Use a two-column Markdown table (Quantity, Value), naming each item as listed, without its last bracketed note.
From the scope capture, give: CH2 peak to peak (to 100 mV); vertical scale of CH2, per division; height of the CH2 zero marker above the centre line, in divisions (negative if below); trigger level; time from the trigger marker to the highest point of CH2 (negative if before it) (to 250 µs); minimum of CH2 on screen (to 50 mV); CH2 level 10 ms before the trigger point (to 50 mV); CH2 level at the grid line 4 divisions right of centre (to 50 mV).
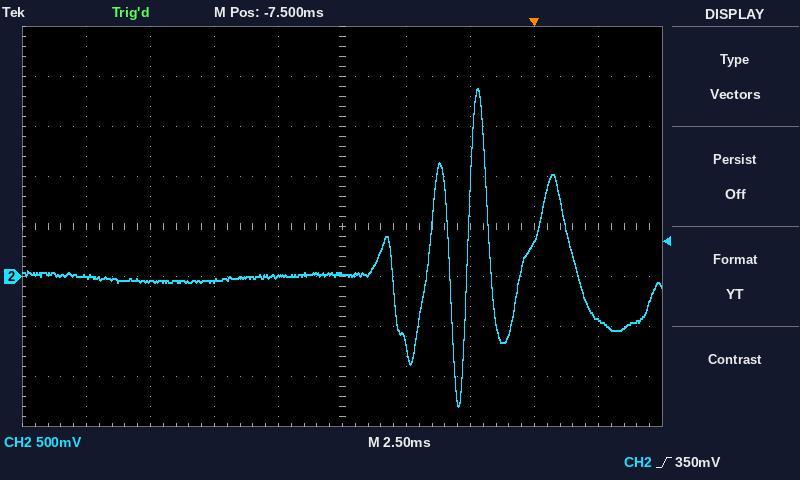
| Quantity | Value |
|---|---|
| CH2 peak to peak | 3.20 V |
| vertical scale of CH2, per division | 500 mV |
| height of the CH2 zero marker above the centre line, in divisions | -1.0 div |
| trigger level | 350 mV |
| time from the trigger marker to the highest point of CH2 (negative if before it) | -2.25 ms |
| minimum of CH2 on screen | -1.30 V |
| CH2 level 10 ms before the trigger point | 0 mV |
| CH2 level at the grid line 4 divisions right of centre | -450 mV |
